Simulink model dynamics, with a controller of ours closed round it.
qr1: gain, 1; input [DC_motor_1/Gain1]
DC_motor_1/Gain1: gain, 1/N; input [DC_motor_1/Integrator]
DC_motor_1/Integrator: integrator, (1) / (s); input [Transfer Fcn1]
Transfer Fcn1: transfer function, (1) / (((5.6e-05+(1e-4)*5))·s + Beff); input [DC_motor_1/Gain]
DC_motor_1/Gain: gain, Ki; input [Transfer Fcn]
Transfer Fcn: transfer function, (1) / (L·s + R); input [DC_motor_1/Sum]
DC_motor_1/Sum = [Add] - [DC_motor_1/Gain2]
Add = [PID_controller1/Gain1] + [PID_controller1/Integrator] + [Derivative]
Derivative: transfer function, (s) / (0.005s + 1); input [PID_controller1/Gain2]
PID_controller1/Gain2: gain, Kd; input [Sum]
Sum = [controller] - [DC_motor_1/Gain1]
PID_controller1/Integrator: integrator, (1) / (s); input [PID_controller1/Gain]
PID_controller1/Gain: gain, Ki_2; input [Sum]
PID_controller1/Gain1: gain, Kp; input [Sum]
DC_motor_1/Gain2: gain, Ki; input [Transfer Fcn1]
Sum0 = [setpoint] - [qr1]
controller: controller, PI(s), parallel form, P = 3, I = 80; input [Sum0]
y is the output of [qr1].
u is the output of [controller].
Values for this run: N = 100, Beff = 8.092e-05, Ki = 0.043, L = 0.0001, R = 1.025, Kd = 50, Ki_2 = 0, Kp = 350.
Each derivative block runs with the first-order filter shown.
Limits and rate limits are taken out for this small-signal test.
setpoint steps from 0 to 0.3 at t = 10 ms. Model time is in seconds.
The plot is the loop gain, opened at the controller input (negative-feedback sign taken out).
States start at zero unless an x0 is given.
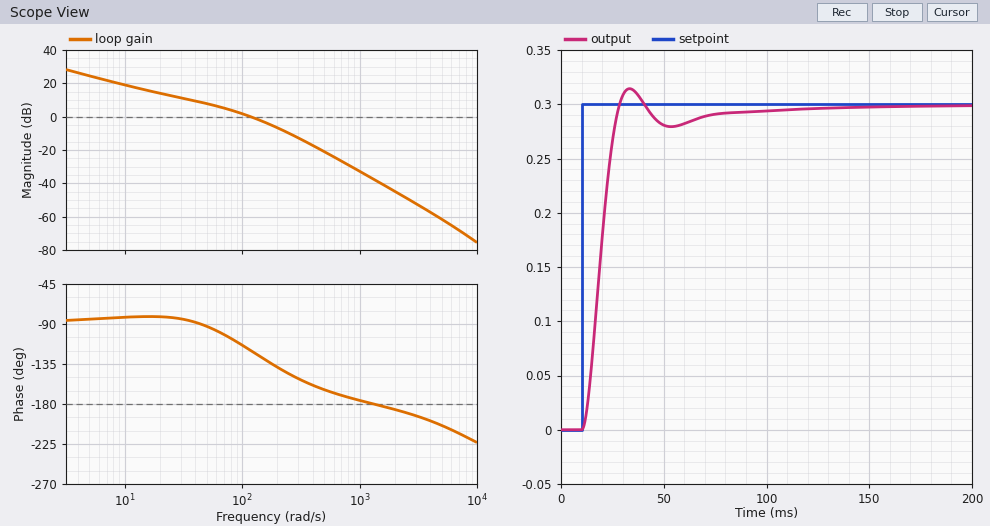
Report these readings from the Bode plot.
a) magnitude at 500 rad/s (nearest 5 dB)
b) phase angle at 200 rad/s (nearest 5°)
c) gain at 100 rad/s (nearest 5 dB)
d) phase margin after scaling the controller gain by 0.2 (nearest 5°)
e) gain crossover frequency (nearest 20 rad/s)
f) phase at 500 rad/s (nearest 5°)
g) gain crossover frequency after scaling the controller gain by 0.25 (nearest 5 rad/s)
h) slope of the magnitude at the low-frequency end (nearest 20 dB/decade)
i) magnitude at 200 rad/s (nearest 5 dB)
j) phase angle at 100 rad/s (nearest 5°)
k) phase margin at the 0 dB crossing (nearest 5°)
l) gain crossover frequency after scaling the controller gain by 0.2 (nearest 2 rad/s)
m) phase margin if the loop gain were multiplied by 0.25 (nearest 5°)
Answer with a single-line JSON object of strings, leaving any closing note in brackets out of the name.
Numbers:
{"magnitude at 500 rad/s": "-20 dB", "phase angle at 200 rad/s": "-140°", "gain at 100 rad/s": "0 dB", "phase margin after scaling the controller gain by 0.2": "100°", "gain crossover frequency": "120 rad/s", "phase at 500 rad/s": "-165°", "gain crossover frequency after scaling the controller gain by 0.25": "25 rad/s", "slope of the magnitude at the low-frequency end": "-20 dB/decade", "magnitude at 200 rad/s": "-5 dB", "phase angle at 100 rad/s": "-115°", "phase margin at the 0 dB crossing": "60°", "gain crossover frequency after scaling the controller gain by 0.2": "20 rad/s", "phase margin if the loop gain were multiplied by 0.25": "95°"}
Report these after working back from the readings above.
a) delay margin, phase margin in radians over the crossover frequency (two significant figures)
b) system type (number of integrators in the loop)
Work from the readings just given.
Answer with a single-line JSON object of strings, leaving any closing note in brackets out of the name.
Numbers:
{"delay margin, phase margin in radians over the crossover frequency": "0.0087 s", "system type": "1"}
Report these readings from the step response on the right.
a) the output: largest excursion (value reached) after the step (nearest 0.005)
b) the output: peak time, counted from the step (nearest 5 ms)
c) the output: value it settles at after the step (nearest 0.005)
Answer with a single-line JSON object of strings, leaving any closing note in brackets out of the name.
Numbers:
{"the output: largest excursion (value reached) after the step": "0.315", "the output: peak time, counted from the step": "25 ms", "the output: value it settles at after the step": "0.300"}
